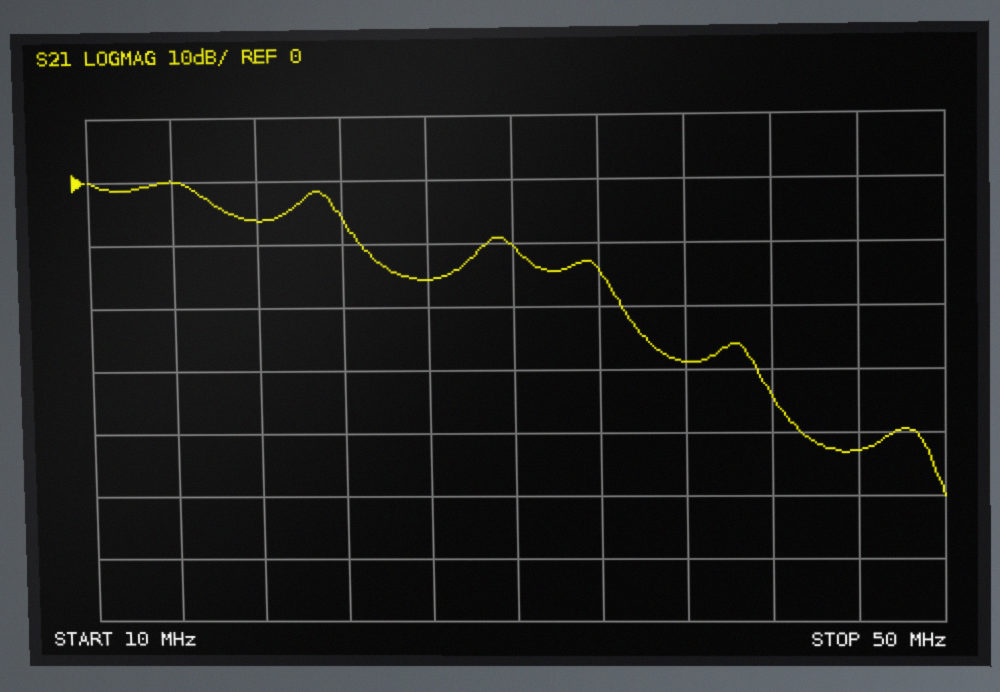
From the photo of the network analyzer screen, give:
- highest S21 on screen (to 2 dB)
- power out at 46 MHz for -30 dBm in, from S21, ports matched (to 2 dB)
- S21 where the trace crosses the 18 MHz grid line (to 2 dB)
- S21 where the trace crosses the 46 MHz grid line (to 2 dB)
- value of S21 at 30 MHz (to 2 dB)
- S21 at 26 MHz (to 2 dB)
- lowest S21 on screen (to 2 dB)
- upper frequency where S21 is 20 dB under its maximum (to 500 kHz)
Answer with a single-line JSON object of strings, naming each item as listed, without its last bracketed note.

{"highest S21 on screen": "0 dB", "power out at 46 MHz for -30 dBm in, from S21, ports matched": "-72 dBm", "S21 where the trace crosses the 18 MHz grid line": "-6 dB", "S21 where the trace crosses the 46 MHz grid line": "-42 dB", "value of S21 at 30 MHz": "-10 dB", "S21 at 26 MHz": "-16 dB", "lowest S21 on screen": "-50 dB", "upper frequency where S21 is 20 dB under its maximum": "35.0 MHz"}
